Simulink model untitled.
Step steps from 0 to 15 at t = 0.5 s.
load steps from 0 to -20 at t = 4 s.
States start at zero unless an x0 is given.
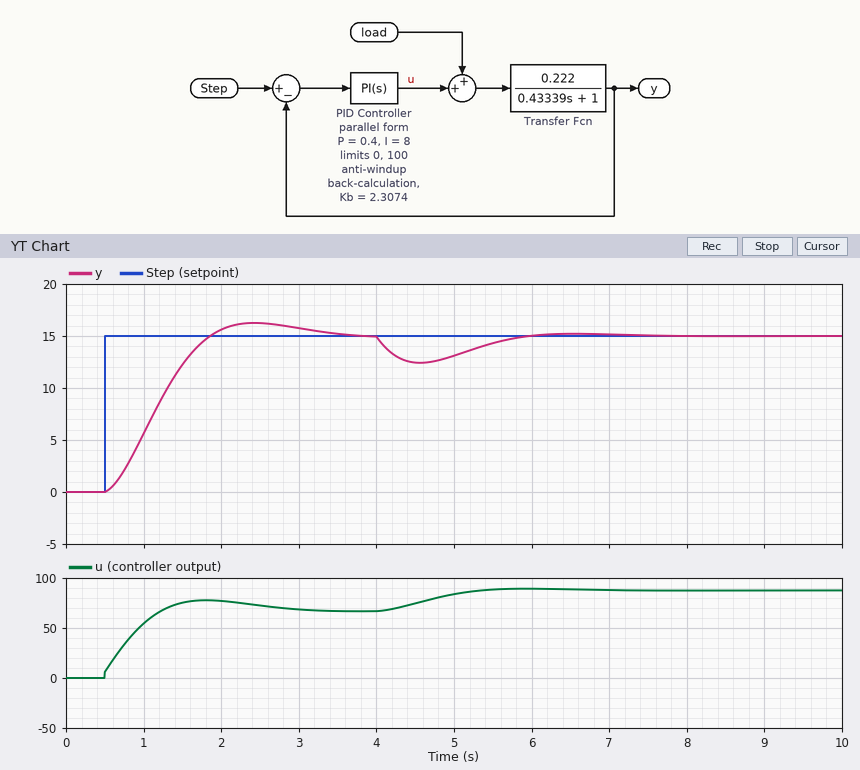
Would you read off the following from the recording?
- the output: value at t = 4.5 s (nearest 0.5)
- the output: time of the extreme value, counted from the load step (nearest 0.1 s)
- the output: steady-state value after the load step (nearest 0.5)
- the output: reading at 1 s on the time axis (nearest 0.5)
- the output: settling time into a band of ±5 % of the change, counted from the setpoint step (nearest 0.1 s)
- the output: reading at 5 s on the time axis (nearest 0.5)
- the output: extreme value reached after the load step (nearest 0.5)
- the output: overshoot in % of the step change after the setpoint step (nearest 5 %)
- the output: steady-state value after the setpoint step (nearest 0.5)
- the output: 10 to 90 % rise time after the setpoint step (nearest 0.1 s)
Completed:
12.5
0.6 s
15.0
5.5
2.5 s
13.0
12.5
10 %
15.0
0.9 s
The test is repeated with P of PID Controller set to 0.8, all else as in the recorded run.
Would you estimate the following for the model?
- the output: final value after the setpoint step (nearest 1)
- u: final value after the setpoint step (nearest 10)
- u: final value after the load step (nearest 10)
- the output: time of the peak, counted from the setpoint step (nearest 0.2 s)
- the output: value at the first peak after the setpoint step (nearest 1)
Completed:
15
70
90
2.0 s
16
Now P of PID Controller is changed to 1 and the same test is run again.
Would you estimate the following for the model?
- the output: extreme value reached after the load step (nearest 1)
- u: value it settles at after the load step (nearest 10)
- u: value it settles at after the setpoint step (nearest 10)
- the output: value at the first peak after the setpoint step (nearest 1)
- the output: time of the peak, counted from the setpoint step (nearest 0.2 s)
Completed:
13
90
70
16
2.0 s
